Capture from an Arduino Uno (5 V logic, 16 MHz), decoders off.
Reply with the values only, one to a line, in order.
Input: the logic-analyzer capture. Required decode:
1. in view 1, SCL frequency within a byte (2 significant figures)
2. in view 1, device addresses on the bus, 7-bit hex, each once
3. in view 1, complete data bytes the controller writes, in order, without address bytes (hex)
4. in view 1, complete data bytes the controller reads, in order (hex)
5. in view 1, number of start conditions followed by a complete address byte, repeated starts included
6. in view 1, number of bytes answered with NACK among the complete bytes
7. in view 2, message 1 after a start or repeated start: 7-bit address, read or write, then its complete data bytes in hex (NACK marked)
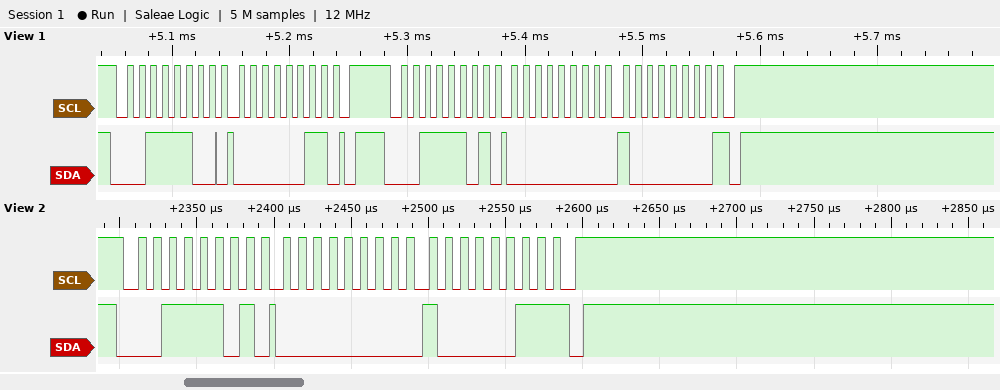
100 kHz
0x1E
03
00 80
2
1
0x1E read: 00 83 NACK
